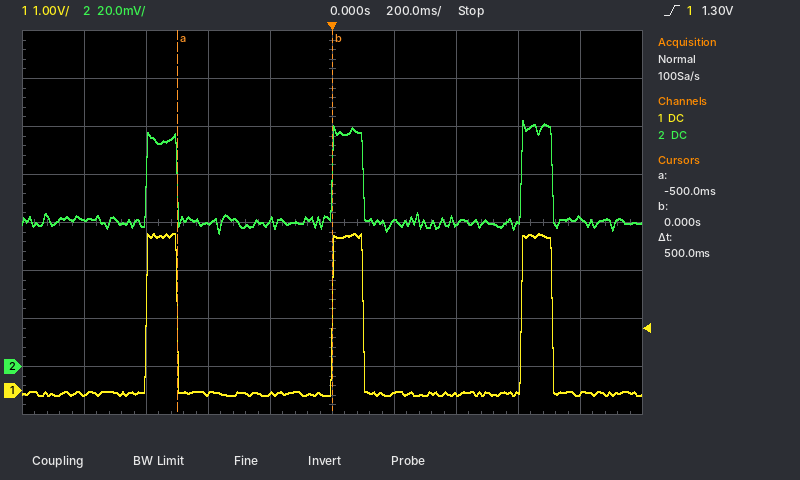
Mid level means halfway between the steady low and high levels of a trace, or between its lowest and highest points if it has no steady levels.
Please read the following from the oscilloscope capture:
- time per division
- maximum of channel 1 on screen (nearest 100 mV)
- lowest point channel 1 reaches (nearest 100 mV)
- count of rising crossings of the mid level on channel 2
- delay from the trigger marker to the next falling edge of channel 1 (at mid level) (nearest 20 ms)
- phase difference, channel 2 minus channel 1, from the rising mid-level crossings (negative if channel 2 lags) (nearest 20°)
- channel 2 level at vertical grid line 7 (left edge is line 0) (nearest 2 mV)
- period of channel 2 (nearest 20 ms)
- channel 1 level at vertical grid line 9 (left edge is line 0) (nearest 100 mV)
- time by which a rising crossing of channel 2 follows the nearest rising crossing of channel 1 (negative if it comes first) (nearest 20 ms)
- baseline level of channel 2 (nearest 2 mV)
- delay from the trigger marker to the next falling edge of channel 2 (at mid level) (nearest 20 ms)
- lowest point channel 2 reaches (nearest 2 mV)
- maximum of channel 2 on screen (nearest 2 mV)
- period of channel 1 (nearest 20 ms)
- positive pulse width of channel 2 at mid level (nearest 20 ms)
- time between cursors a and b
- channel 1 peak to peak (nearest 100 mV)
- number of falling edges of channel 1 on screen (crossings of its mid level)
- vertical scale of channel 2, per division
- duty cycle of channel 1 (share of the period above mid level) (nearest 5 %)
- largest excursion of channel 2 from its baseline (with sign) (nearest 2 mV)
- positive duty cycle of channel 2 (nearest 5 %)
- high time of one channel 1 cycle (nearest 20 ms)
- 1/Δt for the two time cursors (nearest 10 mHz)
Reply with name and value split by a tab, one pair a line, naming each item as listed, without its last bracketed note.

time per division	200 ms
maximum of channel 1 on screen	3.3 V
lowest point channel 1 reaches	-100 mV
count of rising crossings of the mid level on channel 2	3
delay from the trigger marker to the next falling edge of channel 1 (at mid level)	100 ms
phase difference, channel 2 minus channel 1, from the rising mid-level crossings (negative if channel 2 lags)	0°
channel 2 level at vertical grid line 7 (left edge is line 0)	60 mV
period of channel 2	600 ms
channel 1 level at vertical grid line 9 (left edge is line 0)	-100 mV
time by which a rising crossing of channel 2 follows the nearest rising crossing of channel 1 (negative if it comes first)	0 ms
baseline level of channel 2	60 mV
delay from the trigger marker to the next falling edge of channel 2 (at mid level)	100 ms
lowest point channel 2 reaches	56 mV
maximum of channel 2 on screen	102 mV
period of channel 1	600 ms
positive pulse width of channel 2 at mid level	100 ms
time between cursors a and b	500 ms
channel 1 peak to peak	3.4 V
number of falling edges of channel 1 on screen	3
vertical scale of channel 2, per division	20 mV
duty cycle of channel 1 (share of the period above mid level)	15 %
largest excursion of channel 2 from its baseline (with sign)	+42 mV
positive duty cycle of channel 2	15 %
high time of one channel 1 cycle	100 ms
1/Δt for the two time cursors	2.00 Hz
